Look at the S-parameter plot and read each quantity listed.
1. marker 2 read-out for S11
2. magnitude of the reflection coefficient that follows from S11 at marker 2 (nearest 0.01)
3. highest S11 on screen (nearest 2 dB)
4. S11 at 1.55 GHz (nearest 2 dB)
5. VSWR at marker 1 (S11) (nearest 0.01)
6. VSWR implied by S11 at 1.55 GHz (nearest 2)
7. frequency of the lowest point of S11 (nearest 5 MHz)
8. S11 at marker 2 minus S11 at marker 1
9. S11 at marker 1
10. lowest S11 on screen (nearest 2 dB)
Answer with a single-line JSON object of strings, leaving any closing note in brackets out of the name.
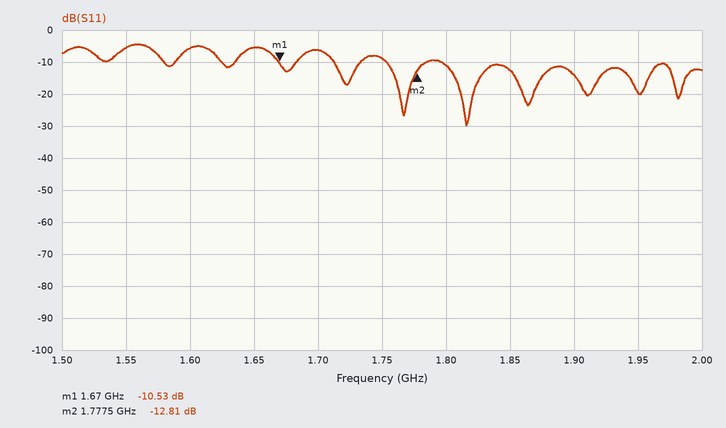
{"marker 2 read-out for S11": "-12.81 dB", "magnitude of the reflection coefficient that follows from S11 at marker 2": "0.23", "highest S11 on screen": "-4 dB", "S11 at 1.55 GHz": "-6 dB", "VSWR at marker 1 (S11)": "1.85", "VSWR implied by S11 at 1.55 GHz": "4", "frequency of the lowest point of S11": "1.815 GHz", "S11 at marker 2 minus S11 at marker 1": "-2.28 dB", "S11 at marker 1": "-10.53 dB", "lowest S11 on screen": "-30 dB"}
